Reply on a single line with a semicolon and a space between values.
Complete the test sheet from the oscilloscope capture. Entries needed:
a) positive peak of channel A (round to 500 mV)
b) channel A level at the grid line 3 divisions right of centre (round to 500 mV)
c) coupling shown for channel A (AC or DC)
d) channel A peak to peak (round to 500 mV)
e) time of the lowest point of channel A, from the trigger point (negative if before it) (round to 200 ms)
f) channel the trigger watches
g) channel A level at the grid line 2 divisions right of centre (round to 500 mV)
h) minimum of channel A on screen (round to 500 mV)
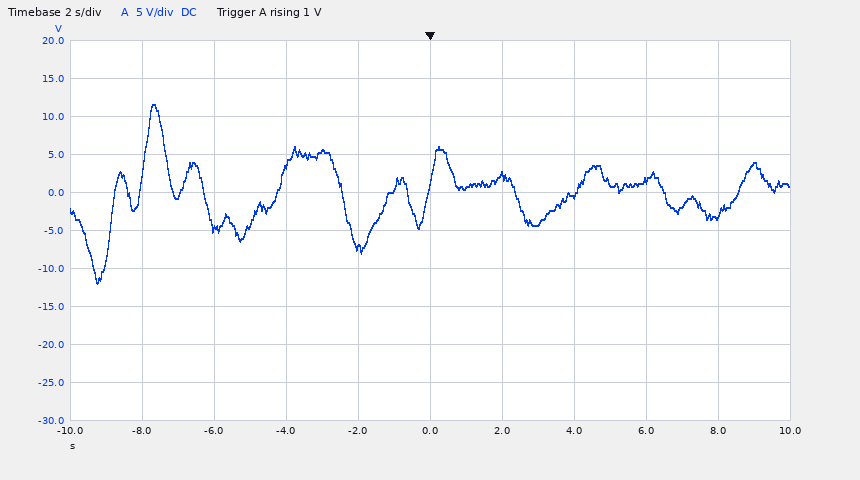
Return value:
11.5 V; 1.5 V; DC; 23.5 V; -9.2 s; channel A; -500 mV; -12.0 V
